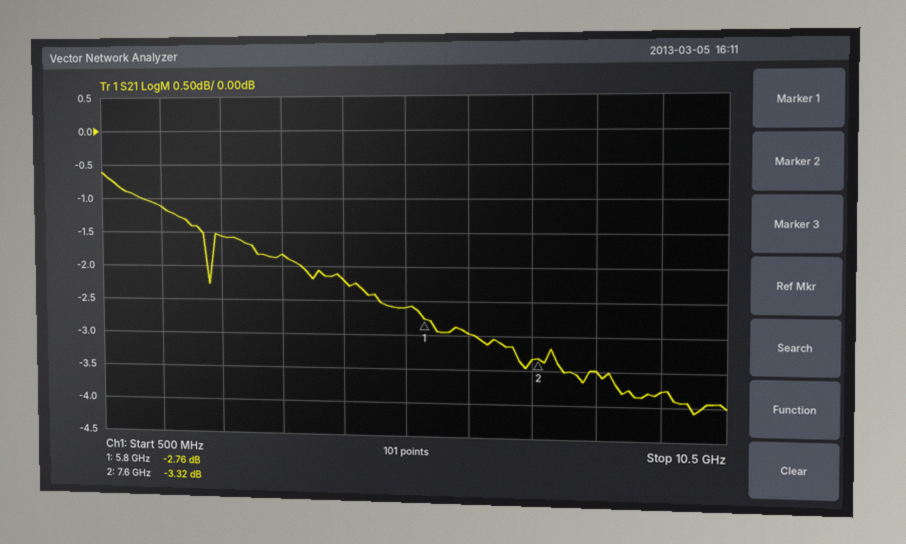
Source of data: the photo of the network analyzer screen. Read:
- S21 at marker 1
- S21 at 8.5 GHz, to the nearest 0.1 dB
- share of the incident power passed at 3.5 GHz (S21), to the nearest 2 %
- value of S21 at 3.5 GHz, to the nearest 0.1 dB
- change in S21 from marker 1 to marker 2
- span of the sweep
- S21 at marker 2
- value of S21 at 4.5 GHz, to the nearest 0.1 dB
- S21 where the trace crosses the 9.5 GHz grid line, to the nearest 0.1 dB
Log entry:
-2.76 dB
-3.5 dB
66 %
-1.8 dB
-0.56 dB
10 GHz
-3.32 dB
-2.2 dB
-3.8 dB
